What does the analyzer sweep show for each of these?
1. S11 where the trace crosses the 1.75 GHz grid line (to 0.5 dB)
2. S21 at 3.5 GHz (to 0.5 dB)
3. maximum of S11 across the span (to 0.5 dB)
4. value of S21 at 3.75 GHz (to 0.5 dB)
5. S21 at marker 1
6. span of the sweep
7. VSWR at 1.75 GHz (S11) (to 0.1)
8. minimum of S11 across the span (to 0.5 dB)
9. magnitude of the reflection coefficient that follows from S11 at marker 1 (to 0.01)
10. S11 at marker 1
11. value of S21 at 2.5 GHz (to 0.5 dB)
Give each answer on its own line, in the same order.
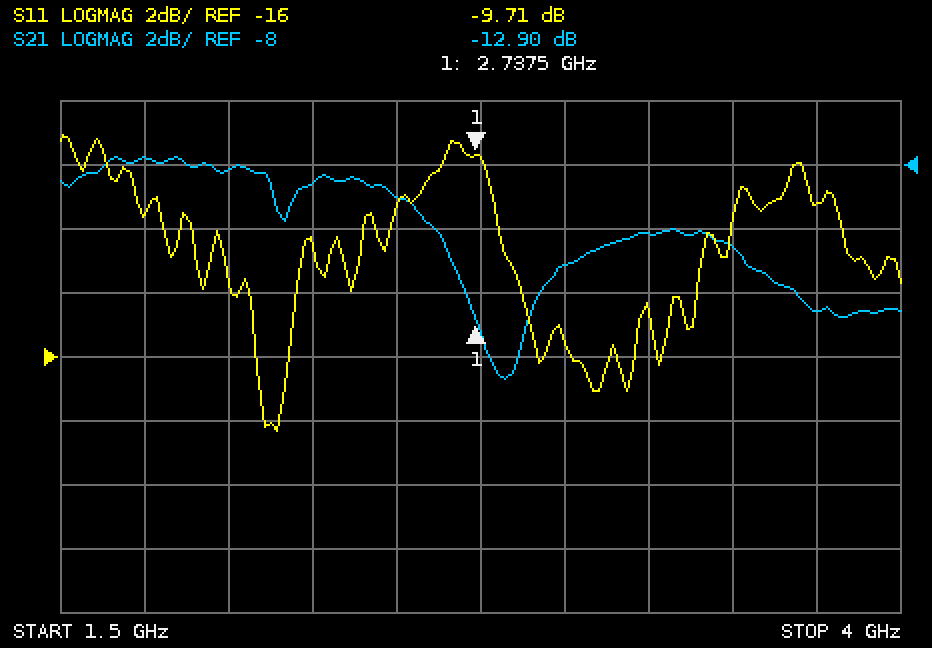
-11.5 dB
-10.5 dB
-9.0 dB
-12.5 dB
-12.90 dB
2.5 GHz
1.7
-18.5 dB
0.33
-9.71 dB
-9.0 dB
